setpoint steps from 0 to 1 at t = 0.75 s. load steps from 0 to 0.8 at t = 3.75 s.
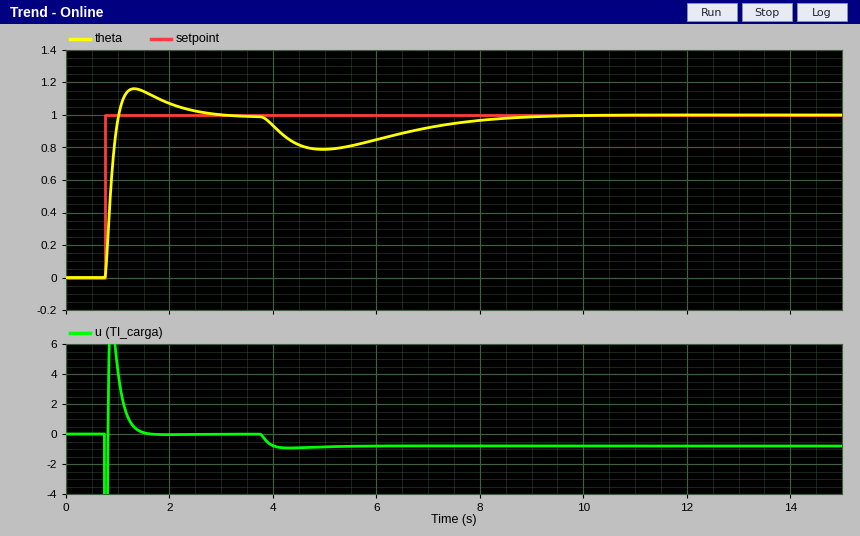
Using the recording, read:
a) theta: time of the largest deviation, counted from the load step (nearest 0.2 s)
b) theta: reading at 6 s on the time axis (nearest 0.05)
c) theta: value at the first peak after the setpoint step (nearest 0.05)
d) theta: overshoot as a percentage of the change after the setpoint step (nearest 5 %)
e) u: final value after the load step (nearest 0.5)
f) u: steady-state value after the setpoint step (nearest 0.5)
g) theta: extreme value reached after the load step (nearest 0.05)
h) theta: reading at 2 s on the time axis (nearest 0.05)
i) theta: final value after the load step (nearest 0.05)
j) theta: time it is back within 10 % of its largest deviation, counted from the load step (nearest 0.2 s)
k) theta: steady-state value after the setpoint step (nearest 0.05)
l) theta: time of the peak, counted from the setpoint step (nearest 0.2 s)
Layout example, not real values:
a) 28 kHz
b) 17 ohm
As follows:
a) 1.2 s
b) 0.85
c) 1.15
d) 15 %
e) -1.0
f) 0.0
g) 0.80
h) 1.05
i) 1.00
j) 4.8 s
k) 1.00
l) 0.6 s
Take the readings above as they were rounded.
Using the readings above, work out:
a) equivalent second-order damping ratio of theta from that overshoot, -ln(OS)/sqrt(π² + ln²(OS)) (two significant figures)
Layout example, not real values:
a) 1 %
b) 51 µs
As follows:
a) 0.52
